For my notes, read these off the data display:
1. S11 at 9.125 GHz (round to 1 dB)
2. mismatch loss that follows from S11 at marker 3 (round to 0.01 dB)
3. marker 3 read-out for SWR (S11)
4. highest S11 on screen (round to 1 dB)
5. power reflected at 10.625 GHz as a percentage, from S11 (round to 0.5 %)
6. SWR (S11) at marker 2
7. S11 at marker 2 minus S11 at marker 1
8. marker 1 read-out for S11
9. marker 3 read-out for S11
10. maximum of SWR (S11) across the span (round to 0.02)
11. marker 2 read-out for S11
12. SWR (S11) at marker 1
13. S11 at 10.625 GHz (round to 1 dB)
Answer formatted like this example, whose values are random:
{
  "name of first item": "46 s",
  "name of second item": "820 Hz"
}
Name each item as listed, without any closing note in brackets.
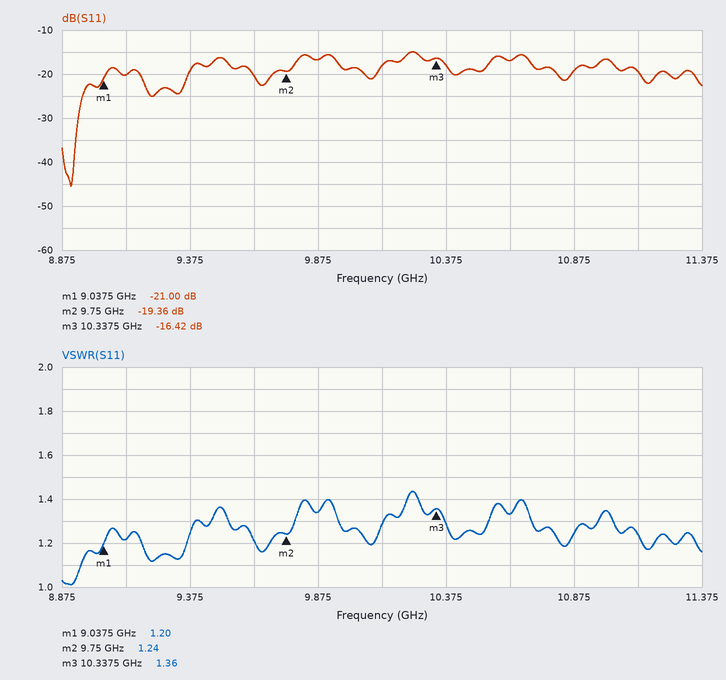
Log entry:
{
  "S11 at 9.125 GHz": "-20 dB",
  "mismatch loss that follows from S11 at marker 3": "0.10 dB",
  "marker 3 read-out for SWR": "1.36",
  "highest S11 on screen": "-15 dB",
  "power reflected at 10.625 GHz as a percentage, from S11": "2.0 %",
  "SWR (S11) at marker 2": "1.24",
  "S11 at marker 2 minus S11 at marker 1": "1.64 dB",
  "marker 1 read-out for S11": "-21.00 dB",
  "marker 3 read-out for S11": "-16.42 dB",
  "maximum of SWR (S11) across the span": "1.44",
  "marker 2 read-out for S11": "-19.36 dB",
  "SWR (S11) at marker 1": "1.20",
  "S11 at 10.625 GHz": "-17 dB"
}
